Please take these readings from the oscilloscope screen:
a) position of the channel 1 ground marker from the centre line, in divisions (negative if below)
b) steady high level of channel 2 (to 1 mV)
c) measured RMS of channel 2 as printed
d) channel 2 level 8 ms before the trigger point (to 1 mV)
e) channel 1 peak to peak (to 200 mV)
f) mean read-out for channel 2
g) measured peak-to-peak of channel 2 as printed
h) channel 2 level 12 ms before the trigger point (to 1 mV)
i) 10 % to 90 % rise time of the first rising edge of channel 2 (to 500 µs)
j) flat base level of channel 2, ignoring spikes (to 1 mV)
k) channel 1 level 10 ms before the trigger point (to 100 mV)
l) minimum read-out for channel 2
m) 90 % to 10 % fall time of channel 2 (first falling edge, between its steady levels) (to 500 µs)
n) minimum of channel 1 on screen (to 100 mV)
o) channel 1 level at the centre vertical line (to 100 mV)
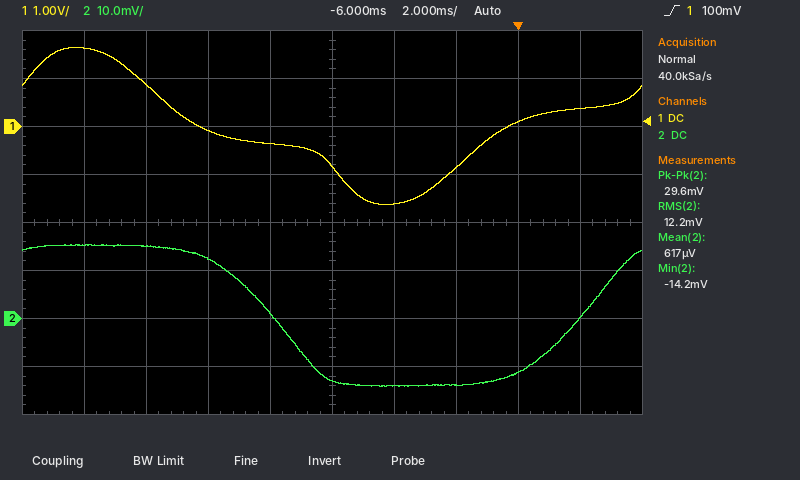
+2.0 div
15 mV
12.2 mV
1 mV
3.2 V
617 µV
29.6 mV
15 mV
3.5 ms
-14 mV
-100 mV
-14.2 mV
3.5 ms
-1.6 V
-800 mV
